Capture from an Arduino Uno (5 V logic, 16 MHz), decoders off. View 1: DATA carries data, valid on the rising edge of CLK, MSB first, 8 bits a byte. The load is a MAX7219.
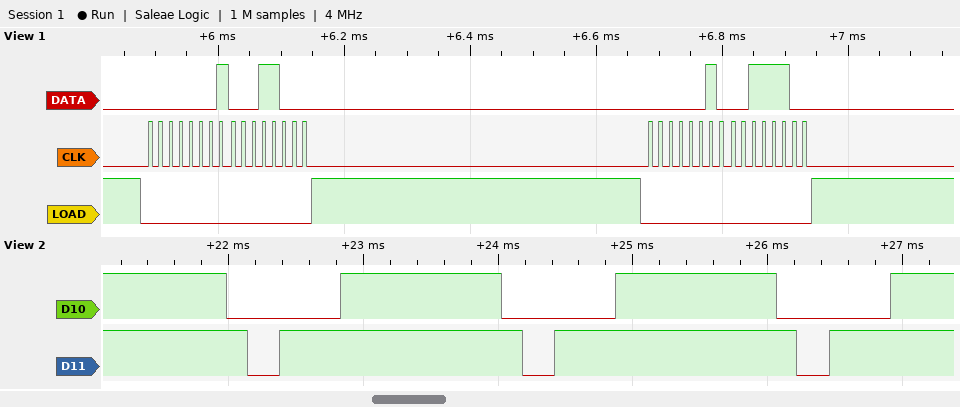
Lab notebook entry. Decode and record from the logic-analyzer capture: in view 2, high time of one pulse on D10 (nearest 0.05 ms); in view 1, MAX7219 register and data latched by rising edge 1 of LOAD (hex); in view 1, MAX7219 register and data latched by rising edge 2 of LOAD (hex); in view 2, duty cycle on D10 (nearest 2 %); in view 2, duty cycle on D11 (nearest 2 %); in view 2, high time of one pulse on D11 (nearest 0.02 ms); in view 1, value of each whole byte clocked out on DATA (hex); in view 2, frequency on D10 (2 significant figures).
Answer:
1.20 ms
register 0x1, data 0x18
register 0x2, data 0x3C
58 %
88 %
1.80 ms
01 18 02 3C
490 Hz
